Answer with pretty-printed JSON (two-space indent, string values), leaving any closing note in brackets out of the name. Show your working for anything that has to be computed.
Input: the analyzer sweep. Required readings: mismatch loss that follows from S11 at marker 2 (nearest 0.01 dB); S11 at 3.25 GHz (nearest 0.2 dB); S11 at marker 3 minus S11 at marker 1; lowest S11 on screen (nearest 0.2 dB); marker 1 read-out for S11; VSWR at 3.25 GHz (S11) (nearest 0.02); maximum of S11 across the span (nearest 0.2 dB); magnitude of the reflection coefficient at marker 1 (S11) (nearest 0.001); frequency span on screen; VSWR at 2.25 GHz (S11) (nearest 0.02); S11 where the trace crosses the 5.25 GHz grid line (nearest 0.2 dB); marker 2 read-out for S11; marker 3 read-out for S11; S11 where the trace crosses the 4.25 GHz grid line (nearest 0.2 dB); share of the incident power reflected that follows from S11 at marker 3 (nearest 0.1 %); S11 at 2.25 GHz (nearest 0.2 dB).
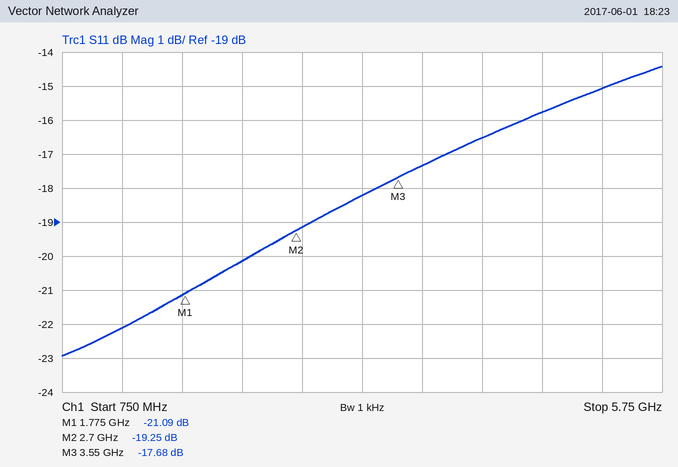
{
  "mismatch loss that follows from S11 at marker 2": "−10 log10(1 − 10^(-19.25/10)) ≈ 0.05 dB",
  "S11 at 3.25 GHz": "-18.2 dB",
  "S11 at marker 3 minus S11 at marker 1": "-17.68 − (-21.09) = 3.41 dB",
  "lowest S11 on screen": "-23.0 dB",
  "marker 1 read-out for S11": "-21.09 dB",
  "VSWR at 3.25 GHz (S11)": "|Γ| = 10^(-18.2/20) = 0.1230; VSWR = (1 + 0.1230)/(1 − 0.1230) ≈ 1.28",
  "maximum of S11 across the span": "-14.4 dB",
  "magnitude of the reflection coefficient at marker 1 (S11)": "10^(-21.09/20) ≈ 0.088",
  "frequency span on screen": "5 GHz",
  "VSWR at 2.25 GHz (S11)": "|Γ| = 10^(-20.2/20) = 0.0977; VSWR = (1 + 0.0977)/(1 − 0.0977) ≈ 1.22",
  "S11 where the trace crosses the 5.25 GHz grid line": "-15.0 dB",
  "marker 2 read-out for S11": "-19.25 dB",
  "marker 3 read-out for S11": "-17.68 dB",
  "S11 where the trace crosses the 4.25 GHz grid line": "-16.6 dB",
  "share of the incident power reflected that follows from S11 at marker 3": "10^(-17.68/10) ≈ 1.7 %",
  "S11 at 2.25 GHz": "-20.2 dB"
}
